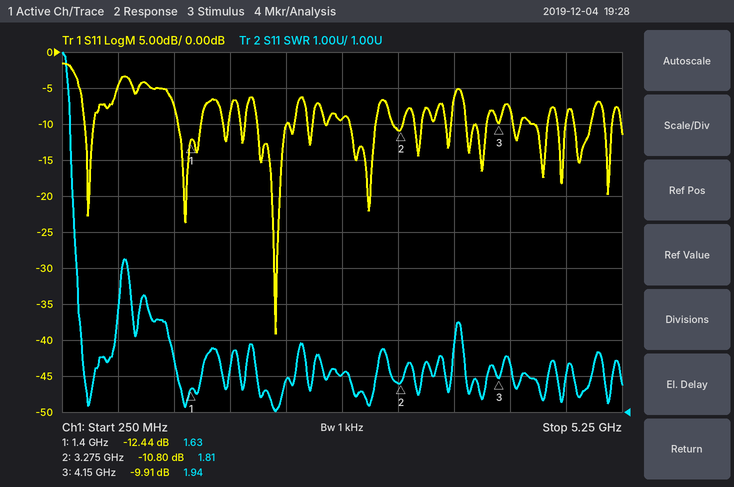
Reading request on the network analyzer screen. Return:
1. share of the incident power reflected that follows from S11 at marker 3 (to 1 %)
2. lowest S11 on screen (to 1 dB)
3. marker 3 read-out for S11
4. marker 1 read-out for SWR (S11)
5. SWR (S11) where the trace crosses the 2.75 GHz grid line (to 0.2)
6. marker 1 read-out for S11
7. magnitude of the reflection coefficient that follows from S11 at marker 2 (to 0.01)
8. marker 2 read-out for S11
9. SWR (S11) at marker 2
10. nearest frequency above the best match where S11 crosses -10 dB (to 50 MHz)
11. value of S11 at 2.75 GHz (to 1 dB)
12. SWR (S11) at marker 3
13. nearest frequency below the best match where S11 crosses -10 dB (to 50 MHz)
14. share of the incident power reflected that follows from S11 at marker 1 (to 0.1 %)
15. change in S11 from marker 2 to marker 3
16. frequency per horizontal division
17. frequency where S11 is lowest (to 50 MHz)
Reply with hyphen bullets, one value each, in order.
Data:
- 10 %
- -39 dB
- -9.91 dB
- 1.63
- 2.0
- -12.44 dB
- 0.29
- -10.80 dB
- 1.81
- 2.25 GHz
- -9 dB
- 1.94
- 2.00 GHz
- 5.7 %
- 0.89 dB
- 500 MHz
- 2.15 GHz
